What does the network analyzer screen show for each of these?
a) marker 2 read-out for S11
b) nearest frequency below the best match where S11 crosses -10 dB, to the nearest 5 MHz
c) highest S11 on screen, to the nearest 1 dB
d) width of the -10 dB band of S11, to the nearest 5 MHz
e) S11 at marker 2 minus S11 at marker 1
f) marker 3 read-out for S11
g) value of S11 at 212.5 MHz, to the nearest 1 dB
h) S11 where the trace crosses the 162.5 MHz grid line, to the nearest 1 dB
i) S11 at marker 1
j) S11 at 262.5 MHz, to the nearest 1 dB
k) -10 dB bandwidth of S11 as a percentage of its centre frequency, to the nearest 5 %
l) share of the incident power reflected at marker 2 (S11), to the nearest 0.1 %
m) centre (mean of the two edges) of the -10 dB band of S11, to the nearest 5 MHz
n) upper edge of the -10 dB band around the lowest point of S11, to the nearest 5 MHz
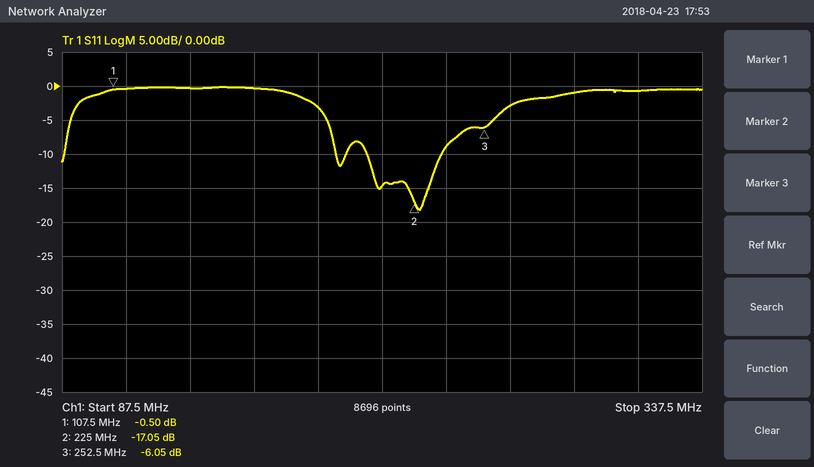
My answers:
-17.05 dB
205 MHz
0 dB
30 MHz
-16.55 dB
-6.05 dB
-15 dB
0 dB
-0.50 dB
-3 dB
15 %
2.0 %
220 MHz
235 MHz
